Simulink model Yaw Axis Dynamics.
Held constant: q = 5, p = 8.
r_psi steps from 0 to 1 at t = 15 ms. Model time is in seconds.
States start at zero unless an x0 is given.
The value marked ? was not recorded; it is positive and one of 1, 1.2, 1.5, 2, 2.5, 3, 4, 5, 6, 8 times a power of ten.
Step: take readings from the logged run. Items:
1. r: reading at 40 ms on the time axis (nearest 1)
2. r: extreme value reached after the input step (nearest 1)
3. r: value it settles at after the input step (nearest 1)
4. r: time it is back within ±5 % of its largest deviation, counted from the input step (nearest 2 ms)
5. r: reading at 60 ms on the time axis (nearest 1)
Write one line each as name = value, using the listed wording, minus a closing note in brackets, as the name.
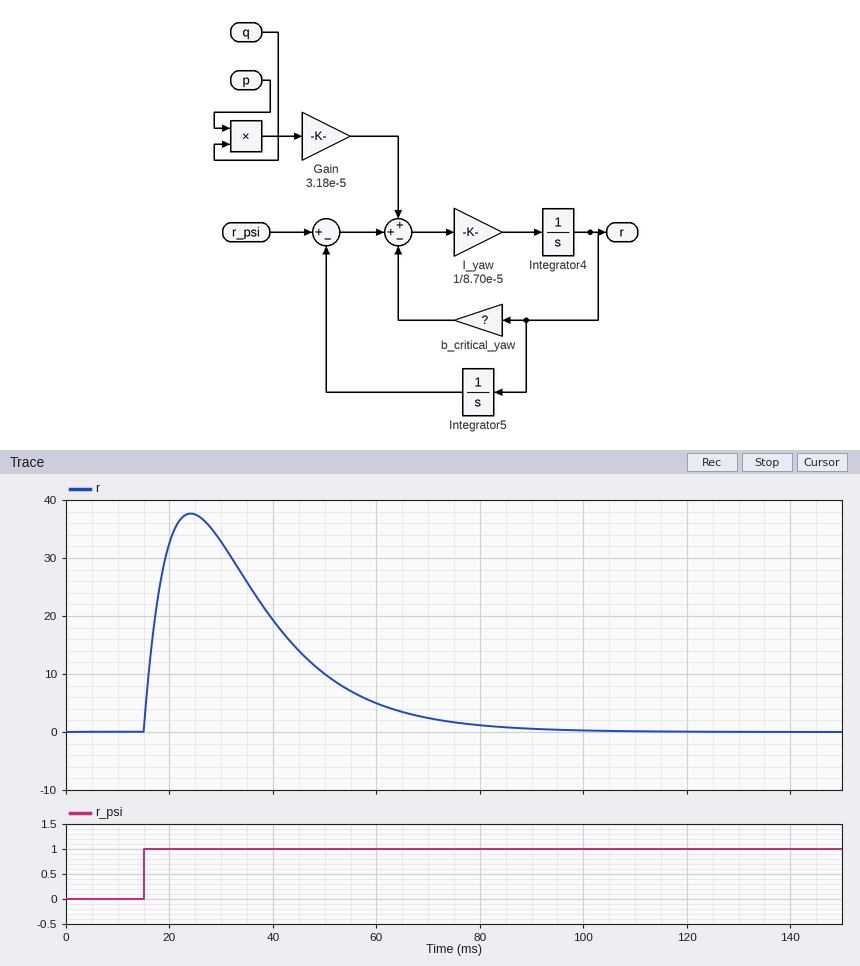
r: reading at 40 ms on the time axis = 19
r: extreme value reached after the input step = 38
r: value it settles at after the input step = 0
r: time it is back within ±5 % of its largest deviation, counted from the input step = 58 ms
r: reading at 60 ms on the time axis = 5
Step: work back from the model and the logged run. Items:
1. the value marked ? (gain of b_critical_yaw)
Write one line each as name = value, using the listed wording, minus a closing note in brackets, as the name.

the value marked ? = 0.02
